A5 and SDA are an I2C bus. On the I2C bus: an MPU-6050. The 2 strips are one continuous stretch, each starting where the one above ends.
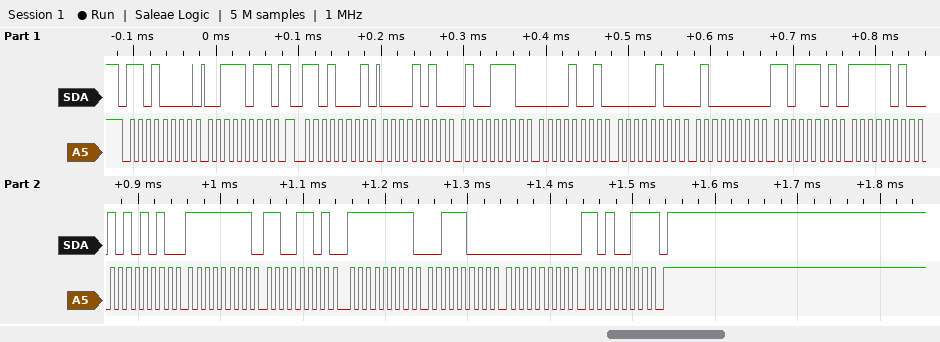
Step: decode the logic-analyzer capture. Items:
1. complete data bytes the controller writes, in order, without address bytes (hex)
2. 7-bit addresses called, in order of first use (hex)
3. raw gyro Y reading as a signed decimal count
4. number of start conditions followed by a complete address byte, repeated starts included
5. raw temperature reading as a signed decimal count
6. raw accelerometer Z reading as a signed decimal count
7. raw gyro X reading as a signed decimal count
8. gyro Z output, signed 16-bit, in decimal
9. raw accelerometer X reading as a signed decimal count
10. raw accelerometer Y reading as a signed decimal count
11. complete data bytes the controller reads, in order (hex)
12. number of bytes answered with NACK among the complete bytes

3B
0x68
-200
2
-1366
16605
-51
211
2638
2308
0A 4E 09 04 40 DD FA AA FF CD FF 38 00 D3
1
